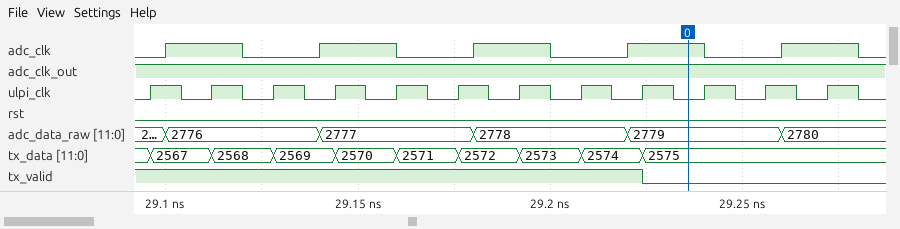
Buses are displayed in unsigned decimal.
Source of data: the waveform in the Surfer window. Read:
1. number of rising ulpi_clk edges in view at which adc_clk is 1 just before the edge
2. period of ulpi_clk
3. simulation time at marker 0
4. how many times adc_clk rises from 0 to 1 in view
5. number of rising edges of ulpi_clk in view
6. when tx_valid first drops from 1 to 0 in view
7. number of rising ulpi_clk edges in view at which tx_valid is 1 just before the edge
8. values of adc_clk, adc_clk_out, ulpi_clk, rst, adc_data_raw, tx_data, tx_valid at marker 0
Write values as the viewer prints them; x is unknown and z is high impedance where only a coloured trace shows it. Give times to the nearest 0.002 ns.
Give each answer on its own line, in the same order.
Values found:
7
0.016 ns
29.236 ns
5
12
29.224 ns
9
adc_clk=1, adc_clk_out=1, ulpi_clk=0, rst=0, adc_data_raw=2779, tx_data=2575, tx_valid=0
